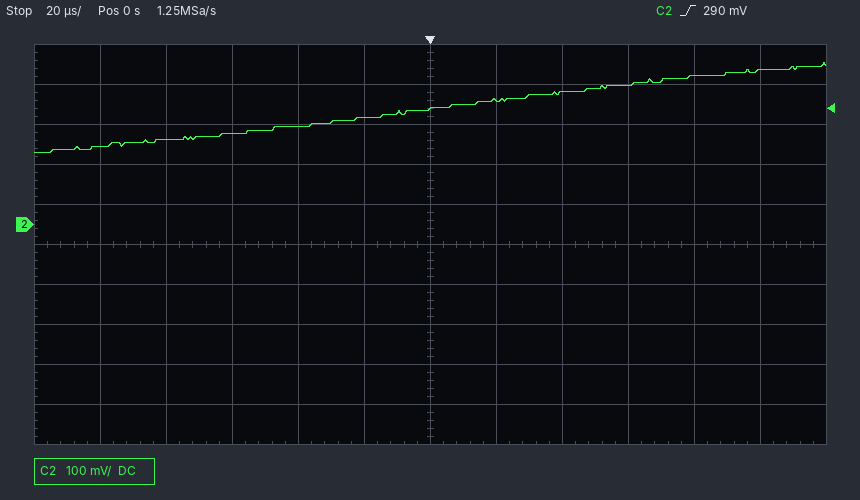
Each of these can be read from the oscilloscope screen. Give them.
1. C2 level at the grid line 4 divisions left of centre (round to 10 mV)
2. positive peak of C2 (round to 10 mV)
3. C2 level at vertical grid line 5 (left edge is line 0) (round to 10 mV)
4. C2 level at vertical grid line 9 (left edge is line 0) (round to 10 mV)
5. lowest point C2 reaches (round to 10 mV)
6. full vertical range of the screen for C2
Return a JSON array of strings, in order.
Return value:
["210 mV", "400 mV", "270 mV", "350 mV", "180 mV", "1 V"]
